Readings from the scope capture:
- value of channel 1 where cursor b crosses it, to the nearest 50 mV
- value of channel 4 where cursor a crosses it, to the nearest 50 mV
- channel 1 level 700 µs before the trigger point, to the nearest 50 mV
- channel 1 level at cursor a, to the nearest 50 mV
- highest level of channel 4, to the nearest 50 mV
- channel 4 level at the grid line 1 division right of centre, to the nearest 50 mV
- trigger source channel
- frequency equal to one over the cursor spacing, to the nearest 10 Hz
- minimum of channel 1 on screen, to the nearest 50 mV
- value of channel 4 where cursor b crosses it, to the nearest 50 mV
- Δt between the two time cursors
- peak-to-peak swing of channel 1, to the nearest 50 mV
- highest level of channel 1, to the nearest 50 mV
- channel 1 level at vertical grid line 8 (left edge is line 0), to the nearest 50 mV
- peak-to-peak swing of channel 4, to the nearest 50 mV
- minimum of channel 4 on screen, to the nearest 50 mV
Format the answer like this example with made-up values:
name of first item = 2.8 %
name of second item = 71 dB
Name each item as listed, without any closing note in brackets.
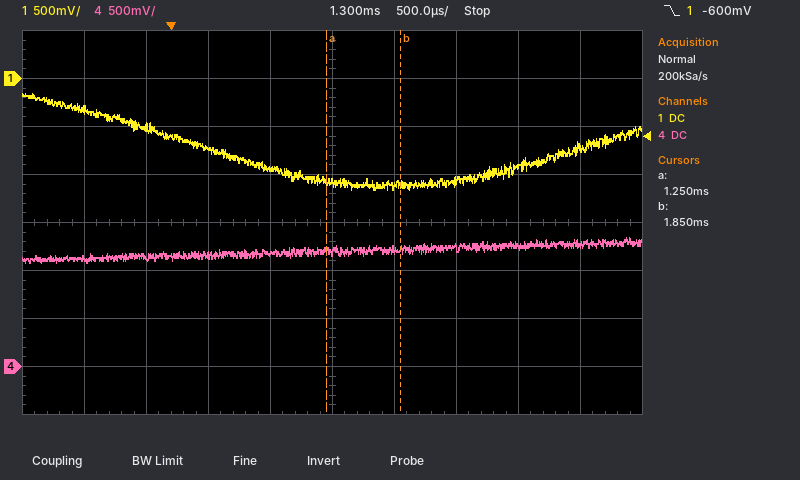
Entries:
value of channel 1 where cursor b crosses it, to the nearest 50 mV = -1.10 V
value of channel 4 where cursor a crosses it, to the nearest 50 mV = 1.20 V
channel 1 level 700 µs before the trigger point, to the nearest 50 mV = -300 mV
channel 1 level at cursor a, to the nearest 50 mV = -1.05 V
highest level of channel 4, to the nearest 50 mV = 1.35 V
channel 4 level at the grid line 1 division right of centre, to the nearest 50 mV = 1.20 V
trigger source channel = channel 1
frequency equal to one over the cursor spacing, to the nearest 10 Hz = 1.67 kHz
minimum of channel 1 on screen, to the nearest 50 mV = -1.15 V
value of channel 4 where cursor b crosses it, to the nearest 50 mV = 1.20 V
Δt between the two time cursors = 600 µs
peak-to-peak swing of channel 1, to the nearest 50 mV = 1.00 V
highest level of channel 1, to the nearest 50 mV = -150 mV
channel 1 level at vertical grid line 8 (left edge is line 0), to the nearest 50 mV = -900 mV
peak-to-peak swing of channel 4, to the nearest 50 mV = 250 mV
minimum of channel 4 on screen, to the nearest 50 mV = 1.10 V
